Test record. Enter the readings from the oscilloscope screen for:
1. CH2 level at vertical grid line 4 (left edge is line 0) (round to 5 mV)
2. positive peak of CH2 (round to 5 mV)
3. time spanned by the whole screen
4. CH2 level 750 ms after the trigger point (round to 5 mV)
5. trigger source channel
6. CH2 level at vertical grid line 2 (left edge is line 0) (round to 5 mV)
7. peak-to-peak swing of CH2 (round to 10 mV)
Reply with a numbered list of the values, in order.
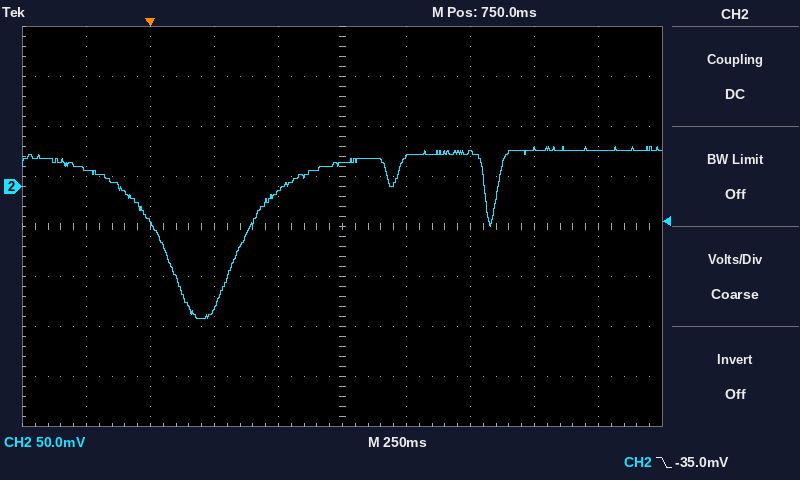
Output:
1. -5 mV
2. 40 mV
3. 2.5 s
4. 25 mV
5. CH2
6. -35 mV
7. 170 mV
